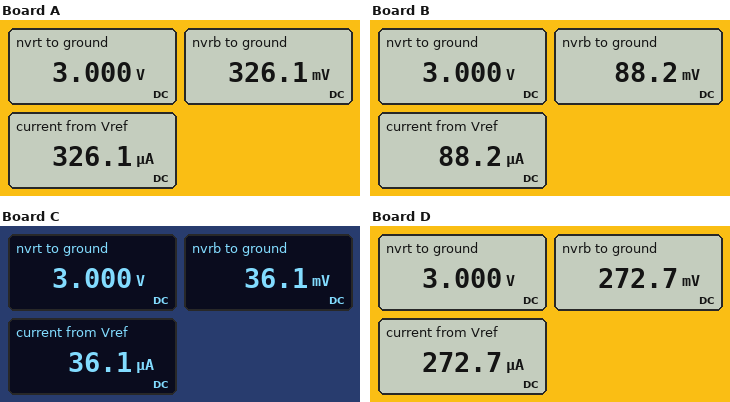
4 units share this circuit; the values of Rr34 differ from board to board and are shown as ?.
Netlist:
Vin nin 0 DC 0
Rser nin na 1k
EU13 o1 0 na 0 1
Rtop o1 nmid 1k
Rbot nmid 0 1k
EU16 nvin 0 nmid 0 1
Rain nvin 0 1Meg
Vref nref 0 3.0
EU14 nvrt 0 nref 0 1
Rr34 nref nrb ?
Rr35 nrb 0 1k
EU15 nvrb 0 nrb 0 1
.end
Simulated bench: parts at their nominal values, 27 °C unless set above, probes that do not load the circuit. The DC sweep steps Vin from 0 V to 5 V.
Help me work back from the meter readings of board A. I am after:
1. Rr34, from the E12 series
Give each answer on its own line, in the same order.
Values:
8.2 kΩ
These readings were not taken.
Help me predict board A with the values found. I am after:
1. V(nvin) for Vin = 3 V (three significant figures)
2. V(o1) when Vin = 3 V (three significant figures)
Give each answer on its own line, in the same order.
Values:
1.50 V
3.00 V
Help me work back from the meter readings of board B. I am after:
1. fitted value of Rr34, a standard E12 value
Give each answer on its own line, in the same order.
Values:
33 kΩ
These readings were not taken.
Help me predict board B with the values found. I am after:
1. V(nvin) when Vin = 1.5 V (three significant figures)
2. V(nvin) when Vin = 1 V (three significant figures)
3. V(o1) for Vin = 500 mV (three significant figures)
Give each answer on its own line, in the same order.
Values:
750 mV
500 mV
500 mV
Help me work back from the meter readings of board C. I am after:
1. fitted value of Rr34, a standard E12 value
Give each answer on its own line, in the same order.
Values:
82 kΩ
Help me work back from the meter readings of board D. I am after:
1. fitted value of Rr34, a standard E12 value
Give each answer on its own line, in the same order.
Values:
10 kΩ
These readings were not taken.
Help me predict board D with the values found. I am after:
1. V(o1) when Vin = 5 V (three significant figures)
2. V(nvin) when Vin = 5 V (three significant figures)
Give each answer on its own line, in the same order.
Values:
5.00 V
2.50 V
